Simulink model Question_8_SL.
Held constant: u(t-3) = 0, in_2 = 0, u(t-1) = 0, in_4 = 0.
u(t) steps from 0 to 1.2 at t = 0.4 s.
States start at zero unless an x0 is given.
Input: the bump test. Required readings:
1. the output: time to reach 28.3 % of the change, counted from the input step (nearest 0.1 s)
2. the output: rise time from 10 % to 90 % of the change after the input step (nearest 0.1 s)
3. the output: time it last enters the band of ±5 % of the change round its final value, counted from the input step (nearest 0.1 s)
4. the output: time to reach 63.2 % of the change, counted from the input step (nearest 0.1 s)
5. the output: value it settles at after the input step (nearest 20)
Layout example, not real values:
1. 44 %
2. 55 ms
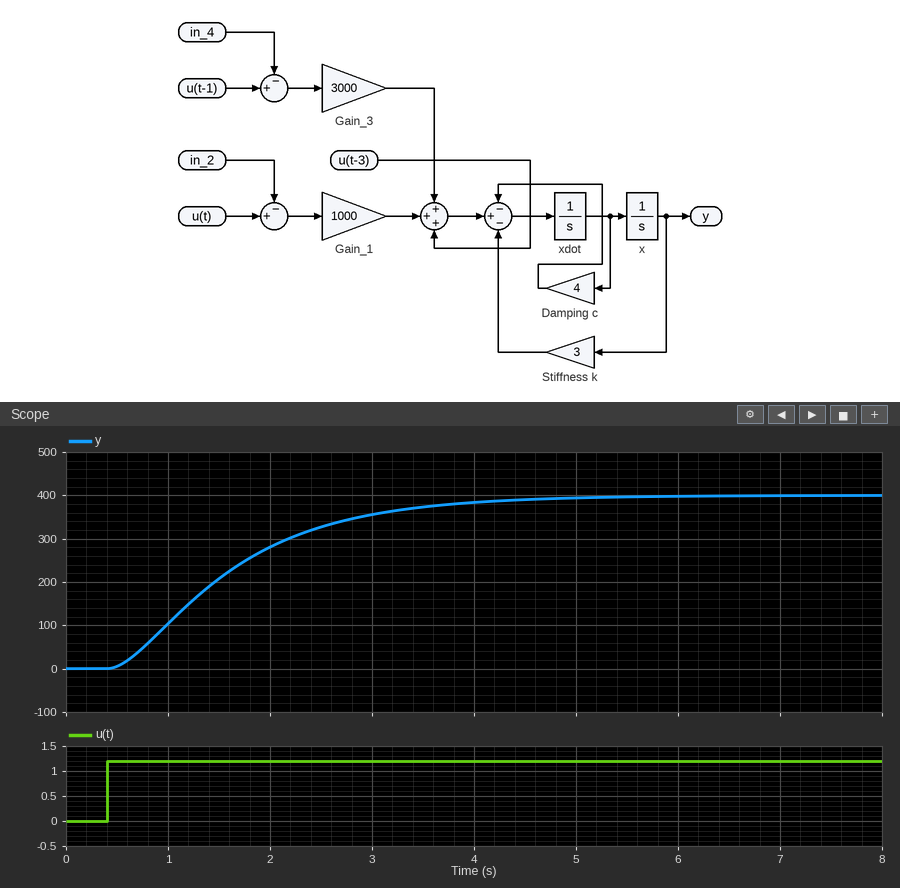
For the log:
1. 0.6 s
2. 2.4 s
3. 3.4 s
4. 1.4 s
5. 400
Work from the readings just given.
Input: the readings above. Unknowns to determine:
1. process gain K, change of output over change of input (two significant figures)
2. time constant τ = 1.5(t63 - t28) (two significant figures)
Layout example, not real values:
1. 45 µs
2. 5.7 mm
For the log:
1. 330
2. 1.2 s
